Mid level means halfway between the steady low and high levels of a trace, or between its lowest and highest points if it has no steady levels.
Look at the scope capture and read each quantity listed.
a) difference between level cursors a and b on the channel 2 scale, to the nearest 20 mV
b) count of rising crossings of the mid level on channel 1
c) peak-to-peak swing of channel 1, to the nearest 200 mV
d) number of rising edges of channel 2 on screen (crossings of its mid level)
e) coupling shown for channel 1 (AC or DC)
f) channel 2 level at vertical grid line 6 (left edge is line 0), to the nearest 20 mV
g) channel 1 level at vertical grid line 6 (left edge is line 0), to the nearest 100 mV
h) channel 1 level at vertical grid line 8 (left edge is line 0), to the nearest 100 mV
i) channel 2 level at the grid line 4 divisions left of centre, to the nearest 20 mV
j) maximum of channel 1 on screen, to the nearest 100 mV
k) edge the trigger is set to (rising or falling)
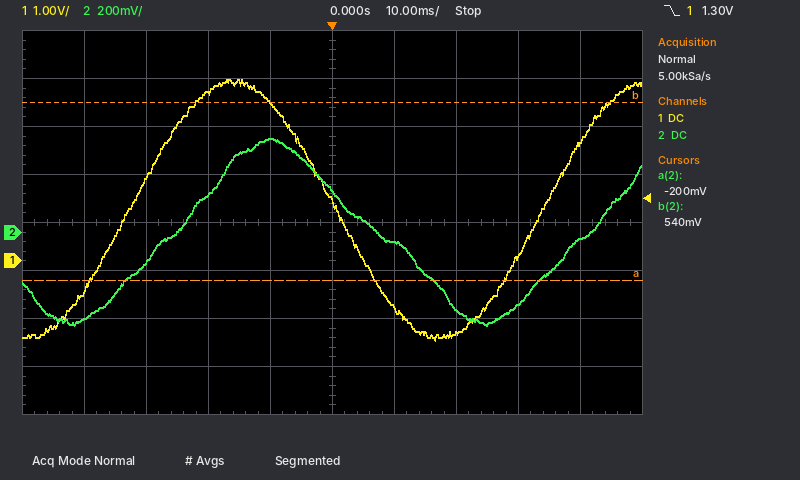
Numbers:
740 mV
2
5.4 V
2
DC
-40 mV
-1.0 V
100 mV
-360 mV
3.8 V
falling
